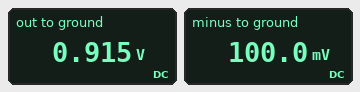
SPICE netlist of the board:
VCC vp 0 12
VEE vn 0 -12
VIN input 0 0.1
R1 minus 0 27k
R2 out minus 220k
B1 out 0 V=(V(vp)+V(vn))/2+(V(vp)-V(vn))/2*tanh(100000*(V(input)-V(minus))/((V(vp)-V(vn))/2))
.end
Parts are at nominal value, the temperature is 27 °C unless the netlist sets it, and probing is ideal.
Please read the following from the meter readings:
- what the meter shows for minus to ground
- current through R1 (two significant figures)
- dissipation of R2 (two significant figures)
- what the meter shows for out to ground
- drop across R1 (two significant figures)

100.0 mV
3.7 µA
3.0 µW
0.915 V
100 mV
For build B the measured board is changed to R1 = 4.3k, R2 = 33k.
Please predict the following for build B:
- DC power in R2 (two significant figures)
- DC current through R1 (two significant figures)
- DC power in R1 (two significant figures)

18 µW
23 µA
2.3 µW
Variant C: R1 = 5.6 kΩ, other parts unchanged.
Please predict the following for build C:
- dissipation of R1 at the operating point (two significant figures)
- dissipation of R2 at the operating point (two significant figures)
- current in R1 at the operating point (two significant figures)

1.8 µW
70 µW
18 µA
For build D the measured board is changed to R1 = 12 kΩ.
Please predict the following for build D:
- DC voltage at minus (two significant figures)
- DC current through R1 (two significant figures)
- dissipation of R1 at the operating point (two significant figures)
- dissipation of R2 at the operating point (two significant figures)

100 mV
8.3 µA
830 nW
15 µW
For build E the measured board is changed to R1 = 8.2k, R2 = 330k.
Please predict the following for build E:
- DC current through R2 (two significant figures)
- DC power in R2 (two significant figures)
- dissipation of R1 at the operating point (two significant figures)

12 µA
49 µW
1.2 µW
